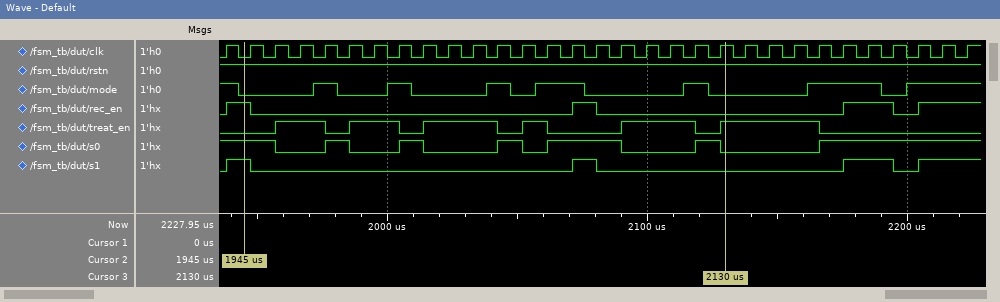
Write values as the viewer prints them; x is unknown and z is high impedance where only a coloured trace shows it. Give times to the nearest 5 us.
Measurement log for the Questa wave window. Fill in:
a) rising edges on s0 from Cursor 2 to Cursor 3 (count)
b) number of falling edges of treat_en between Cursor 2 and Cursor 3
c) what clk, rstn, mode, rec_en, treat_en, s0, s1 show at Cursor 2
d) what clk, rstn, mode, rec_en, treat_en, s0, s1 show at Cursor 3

5
5
clk=0, rstn=1, mode=0, rec_en=1, treat_en=0, s0=1, s1=1
clk=1, rstn=1, mode=0, rec_en=0, treat_en=1, s0=0, s1=0
